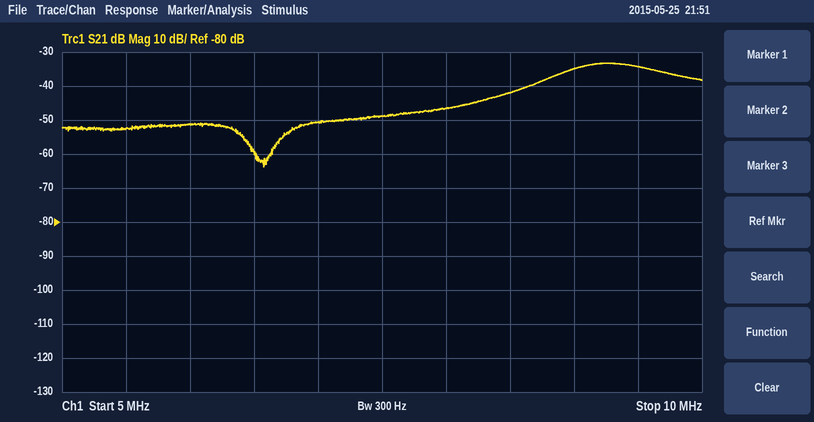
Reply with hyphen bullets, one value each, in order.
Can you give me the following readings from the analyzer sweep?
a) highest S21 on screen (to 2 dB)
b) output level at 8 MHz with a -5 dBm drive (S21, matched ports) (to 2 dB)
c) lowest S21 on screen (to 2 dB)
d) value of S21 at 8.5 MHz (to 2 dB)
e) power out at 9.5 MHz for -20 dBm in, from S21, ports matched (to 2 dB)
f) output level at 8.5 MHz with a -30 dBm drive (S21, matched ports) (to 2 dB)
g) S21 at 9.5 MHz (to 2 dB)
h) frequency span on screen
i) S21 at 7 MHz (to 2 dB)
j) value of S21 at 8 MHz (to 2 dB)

- -34 dB
- -52 dBm
- -64 dB
- -42 dB
- -54 dBm
- -72 dBm
- -34 dB
- 5 MHz
- -50 dB
- -46 dB
